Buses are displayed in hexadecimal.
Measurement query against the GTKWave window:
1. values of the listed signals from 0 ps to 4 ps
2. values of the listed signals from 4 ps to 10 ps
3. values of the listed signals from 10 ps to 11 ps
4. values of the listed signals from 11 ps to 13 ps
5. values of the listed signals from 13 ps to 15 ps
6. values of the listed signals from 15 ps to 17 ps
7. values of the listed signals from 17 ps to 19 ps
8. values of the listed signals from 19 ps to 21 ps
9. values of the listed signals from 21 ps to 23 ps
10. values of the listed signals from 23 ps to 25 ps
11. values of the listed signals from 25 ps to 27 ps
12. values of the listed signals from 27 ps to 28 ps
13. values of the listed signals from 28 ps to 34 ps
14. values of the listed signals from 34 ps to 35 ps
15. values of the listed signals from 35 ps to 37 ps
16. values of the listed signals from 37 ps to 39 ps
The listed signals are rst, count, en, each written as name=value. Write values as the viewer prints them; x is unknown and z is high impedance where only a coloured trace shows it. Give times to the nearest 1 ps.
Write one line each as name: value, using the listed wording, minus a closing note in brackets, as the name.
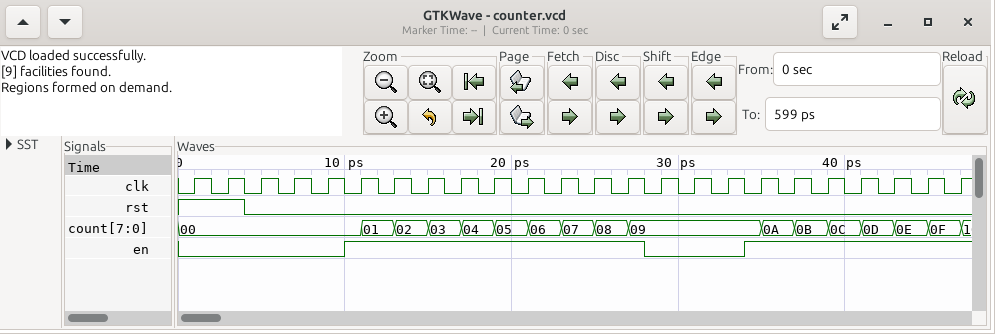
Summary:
values of the listed signals from 0 ps to 4 ps: rst=1, count=00, en=0
values of the listed signals from 4 ps to 10 ps: rst=0, count=00, en=0
values of the listed signals from 10 ps to 11 ps: rst=0, count=00, en=1
values of the listed signals from 11 ps to 13 ps: rst=0, count=01, en=1
values of the listed signals from 13 ps to 15 ps: rst=0, count=02, en=1
values of the listed signals from 15 ps to 17 ps: rst=0, count=03, en=1
values of the listed signals from 17 ps to 19 ps: rst=0, count=04, en=1
values of the listed signals from 19 ps to 21 ps: rst=0, count=05, en=1
values of the listed signals from 21 ps to 23 ps: rst=0, count=06, en=1
values of the listed signals from 23 ps to 25 ps: rst=0, count=07, en=1
values of the listed signals from 25 ps to 27 ps: rst=0, count=08, en=1
values of the listed signals from 27 ps to 28 ps: rst=0, count=09, en=1
values of the listed signals from 28 ps to 34 ps: rst=0, count=09, en=0
values of the listed signals from 34 ps to 35 ps: rst=0, count=09, en=1
values of the listed signals from 35 ps to 37 ps: rst=0, count=0A, en=1
values of the listed signals from 37 ps to 39 ps: rst=0, count=0B, en=1
